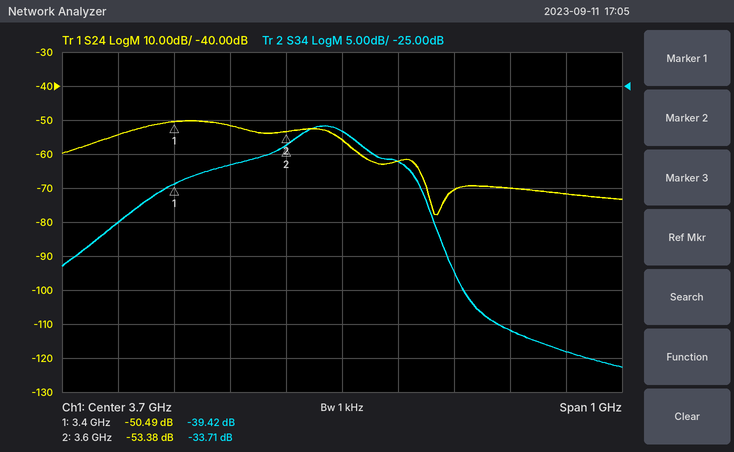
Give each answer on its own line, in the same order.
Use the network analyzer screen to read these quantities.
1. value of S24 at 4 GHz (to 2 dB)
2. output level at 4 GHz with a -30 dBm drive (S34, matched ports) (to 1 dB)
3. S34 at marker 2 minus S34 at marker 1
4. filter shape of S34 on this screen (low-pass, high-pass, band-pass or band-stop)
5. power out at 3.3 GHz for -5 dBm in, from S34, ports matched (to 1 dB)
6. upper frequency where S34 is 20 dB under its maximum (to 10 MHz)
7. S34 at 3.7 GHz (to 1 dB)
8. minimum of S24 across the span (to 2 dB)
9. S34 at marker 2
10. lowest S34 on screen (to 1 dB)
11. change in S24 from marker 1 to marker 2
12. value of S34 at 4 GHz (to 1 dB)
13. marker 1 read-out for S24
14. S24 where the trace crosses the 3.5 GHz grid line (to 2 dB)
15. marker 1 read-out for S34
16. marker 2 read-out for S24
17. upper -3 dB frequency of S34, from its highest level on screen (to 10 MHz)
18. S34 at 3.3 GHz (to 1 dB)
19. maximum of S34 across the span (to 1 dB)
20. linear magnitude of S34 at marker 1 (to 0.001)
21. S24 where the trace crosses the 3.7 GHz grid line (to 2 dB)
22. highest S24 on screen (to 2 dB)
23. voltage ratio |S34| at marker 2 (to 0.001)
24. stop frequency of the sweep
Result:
-70 dB
-91 dBm
5.71 dB
band-pass
-50 dBm
3.89 GHz
-32 dB
-78 dB
-33.71 dB
-66 dB
-2.89 dB
-61 dB
-50.49 dB
-52 dB
-39.42 dB
-53.38 dB
3.74 GHz
-45 dB
-31 dB
0.011
-56 dB
-50 dB
0.021
4.2 GHz
